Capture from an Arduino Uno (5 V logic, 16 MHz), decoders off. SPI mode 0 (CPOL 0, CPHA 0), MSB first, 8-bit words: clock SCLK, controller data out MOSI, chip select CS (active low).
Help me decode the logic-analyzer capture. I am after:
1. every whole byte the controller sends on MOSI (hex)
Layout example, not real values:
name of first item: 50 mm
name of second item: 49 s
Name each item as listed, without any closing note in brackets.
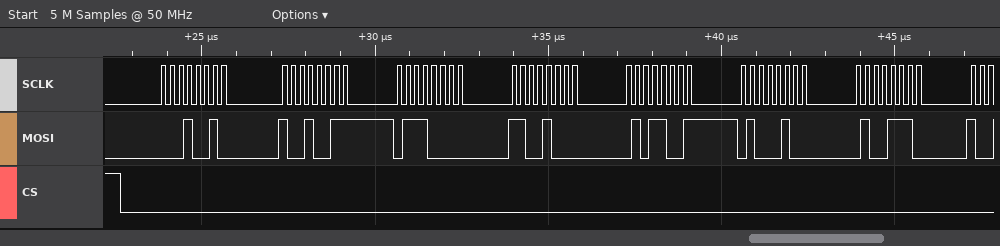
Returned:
every whole byte the controller sends on MOSI: 12 93 70 C8 59 44 4E
